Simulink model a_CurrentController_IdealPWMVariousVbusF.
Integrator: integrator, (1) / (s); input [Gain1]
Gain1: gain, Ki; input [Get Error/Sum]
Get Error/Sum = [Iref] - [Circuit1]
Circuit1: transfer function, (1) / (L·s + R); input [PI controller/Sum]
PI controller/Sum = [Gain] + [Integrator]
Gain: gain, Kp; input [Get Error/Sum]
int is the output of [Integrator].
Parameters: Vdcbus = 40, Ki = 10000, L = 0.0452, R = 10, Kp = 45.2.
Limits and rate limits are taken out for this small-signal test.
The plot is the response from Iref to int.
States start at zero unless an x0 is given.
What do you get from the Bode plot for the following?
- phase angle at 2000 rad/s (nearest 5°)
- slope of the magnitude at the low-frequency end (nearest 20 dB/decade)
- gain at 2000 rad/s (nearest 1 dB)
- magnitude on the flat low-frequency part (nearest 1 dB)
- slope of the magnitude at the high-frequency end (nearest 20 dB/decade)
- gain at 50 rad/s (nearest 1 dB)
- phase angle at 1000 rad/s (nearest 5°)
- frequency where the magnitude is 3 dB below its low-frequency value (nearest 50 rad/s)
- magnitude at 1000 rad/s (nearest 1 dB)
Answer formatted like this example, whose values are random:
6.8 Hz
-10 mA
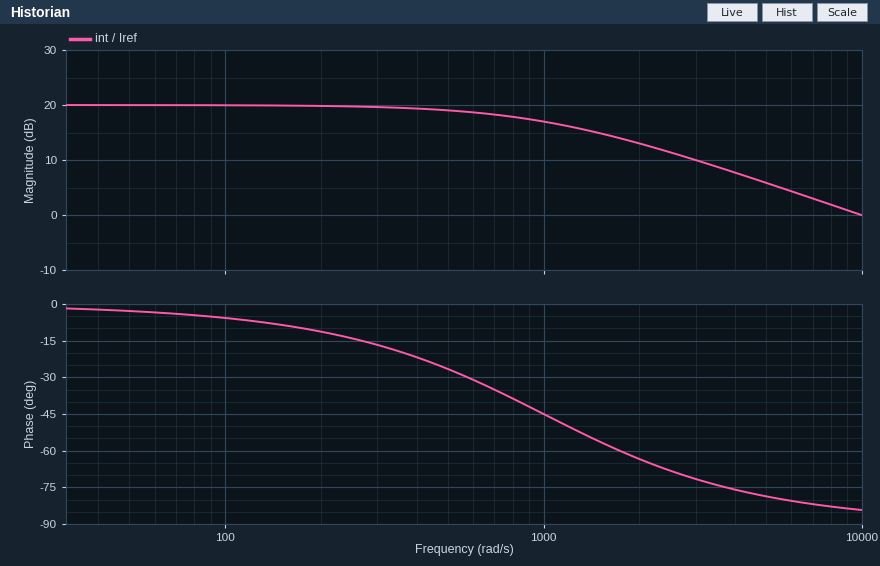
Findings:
-65°
0 dB/decade
13 dB
20 dB
-20 dB/decade
20 dB
-45°
1000 rad/s
17 dB
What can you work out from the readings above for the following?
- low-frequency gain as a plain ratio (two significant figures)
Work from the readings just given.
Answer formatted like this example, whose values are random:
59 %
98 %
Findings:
10
